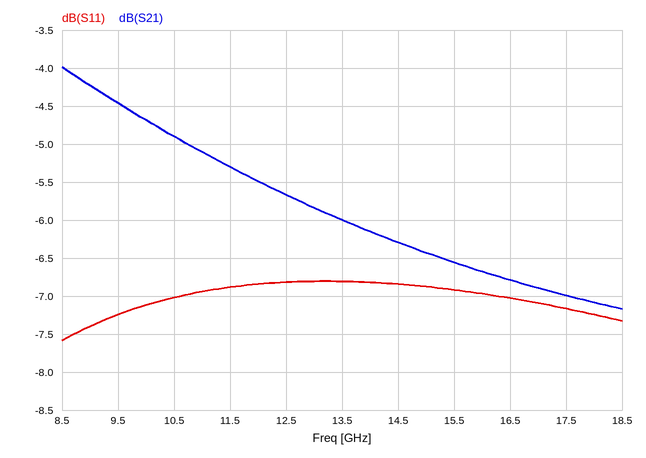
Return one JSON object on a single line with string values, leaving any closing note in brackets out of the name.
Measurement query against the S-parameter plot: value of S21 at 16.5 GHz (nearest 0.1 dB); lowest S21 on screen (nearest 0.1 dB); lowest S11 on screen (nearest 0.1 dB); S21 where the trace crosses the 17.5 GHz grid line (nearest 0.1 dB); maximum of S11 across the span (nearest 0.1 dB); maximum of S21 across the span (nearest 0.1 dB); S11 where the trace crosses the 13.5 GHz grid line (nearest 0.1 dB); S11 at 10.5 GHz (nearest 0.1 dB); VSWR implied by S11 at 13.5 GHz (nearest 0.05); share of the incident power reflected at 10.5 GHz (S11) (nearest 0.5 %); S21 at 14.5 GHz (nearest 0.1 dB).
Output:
{"value of S21 at 16.5 GHz": "-6.8 dB", "lowest S21 on screen": "-7.2 dB", "lowest S11 on screen": "-7.6 dB", "S21 where the trace crosses the 17.5 GHz grid line": "-7.0 dB", "maximum of S11 across the span": "-6.8 dB", "maximum of S21 across the span": "-4.0 dB", "S11 where the trace crosses the 13.5 GHz grid line": "-6.8 dB", "S11 at 10.5 GHz": "-7.0 dB", "VSWR implied by S11 at 13.5 GHz": "2.70", "share of the incident power reflected at 10.5 GHz (S11)": "20.0 %", "S21 at 14.5 GHz": "-6.3 dB"}
